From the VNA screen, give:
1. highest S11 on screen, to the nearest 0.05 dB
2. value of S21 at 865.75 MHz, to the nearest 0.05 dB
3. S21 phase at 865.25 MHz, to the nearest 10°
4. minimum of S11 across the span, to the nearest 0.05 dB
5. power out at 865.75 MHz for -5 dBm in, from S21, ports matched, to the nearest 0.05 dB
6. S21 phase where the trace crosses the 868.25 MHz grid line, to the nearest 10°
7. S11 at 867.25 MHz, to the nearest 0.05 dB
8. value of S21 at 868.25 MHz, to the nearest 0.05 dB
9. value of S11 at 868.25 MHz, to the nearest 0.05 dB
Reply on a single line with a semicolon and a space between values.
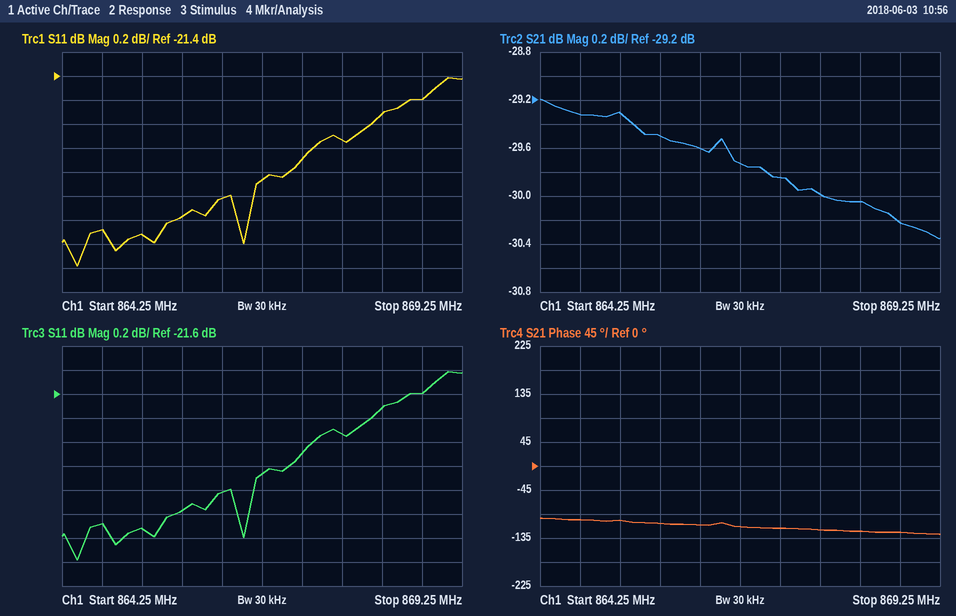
-21.40 dB; -29.50 dB; -100°; -23.00 dB; -34.50 dBm; -120°; -22.10 dB; -30.05 dB; -21.70 dB
